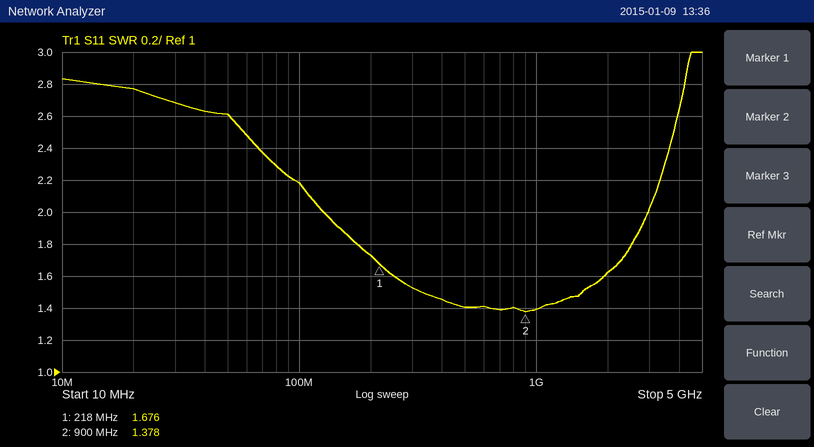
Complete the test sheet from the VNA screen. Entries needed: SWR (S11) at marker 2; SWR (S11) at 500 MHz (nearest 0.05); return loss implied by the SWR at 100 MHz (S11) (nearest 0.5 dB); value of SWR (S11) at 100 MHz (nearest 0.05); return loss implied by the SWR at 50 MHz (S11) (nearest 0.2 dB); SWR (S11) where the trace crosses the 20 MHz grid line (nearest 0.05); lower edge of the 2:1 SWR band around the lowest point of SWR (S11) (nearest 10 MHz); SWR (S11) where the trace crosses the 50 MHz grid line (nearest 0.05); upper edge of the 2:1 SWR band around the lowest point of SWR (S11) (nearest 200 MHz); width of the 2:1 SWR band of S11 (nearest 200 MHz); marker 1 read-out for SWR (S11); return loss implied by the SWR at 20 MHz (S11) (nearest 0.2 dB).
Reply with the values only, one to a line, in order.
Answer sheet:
1.378
1.40
8.5 dB
2.20
7.0 dB
2.75
130 MHz
2.60
3.0 GHz
2.8 GHz
1.676
6.6 dB
